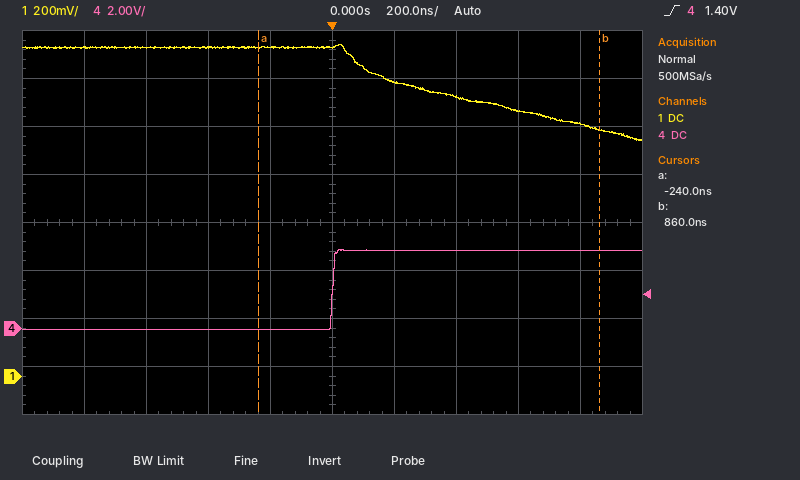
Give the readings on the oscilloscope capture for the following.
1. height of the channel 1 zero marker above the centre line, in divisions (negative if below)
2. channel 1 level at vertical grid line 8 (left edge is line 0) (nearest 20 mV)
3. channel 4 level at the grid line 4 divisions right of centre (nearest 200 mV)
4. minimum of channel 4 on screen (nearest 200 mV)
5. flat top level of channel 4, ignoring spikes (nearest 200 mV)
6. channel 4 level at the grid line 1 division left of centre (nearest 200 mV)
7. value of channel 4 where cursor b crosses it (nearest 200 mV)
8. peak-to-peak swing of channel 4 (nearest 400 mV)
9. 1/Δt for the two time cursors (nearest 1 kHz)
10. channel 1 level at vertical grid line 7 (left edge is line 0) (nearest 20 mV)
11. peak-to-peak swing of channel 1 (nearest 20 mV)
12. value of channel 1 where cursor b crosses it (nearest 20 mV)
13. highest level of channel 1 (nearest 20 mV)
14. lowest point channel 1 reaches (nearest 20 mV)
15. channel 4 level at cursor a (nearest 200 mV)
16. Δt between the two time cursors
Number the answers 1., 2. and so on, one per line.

1. -3.2 div
2. 1.10 V
3. 3.2 V
4. 0.0 V
5. 3.2 V
6. 0.0 V
7. 3.2 V
8. 3.2 V
9. 909 kHz
10. 1.16 V
11. 400 mV
12. 1.02 V
13. 1.38 V
14. 980 mV
15. 0.0 V
16. 1.10 µs
